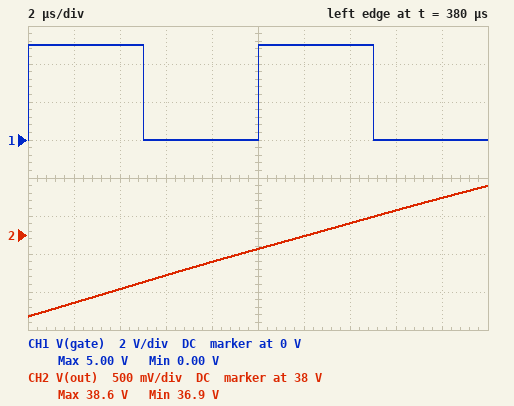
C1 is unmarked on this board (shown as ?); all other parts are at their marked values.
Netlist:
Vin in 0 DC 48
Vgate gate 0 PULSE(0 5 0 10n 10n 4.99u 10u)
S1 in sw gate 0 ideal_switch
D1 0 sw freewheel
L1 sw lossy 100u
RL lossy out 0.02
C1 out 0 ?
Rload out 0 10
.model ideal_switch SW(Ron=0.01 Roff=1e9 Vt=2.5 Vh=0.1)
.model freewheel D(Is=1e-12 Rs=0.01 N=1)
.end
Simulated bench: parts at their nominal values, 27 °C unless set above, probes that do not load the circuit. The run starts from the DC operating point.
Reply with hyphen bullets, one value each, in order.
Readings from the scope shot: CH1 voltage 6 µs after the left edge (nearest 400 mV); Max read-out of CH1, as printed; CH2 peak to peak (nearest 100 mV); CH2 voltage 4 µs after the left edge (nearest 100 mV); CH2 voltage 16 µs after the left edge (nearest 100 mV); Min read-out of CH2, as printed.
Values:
- 0 V
- 5.00 V
- 1.7 V
- 37.3 V
- 38.3 V
- 36.9 V
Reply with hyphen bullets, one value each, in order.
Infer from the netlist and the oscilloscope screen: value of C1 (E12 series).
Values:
- 270 µF
